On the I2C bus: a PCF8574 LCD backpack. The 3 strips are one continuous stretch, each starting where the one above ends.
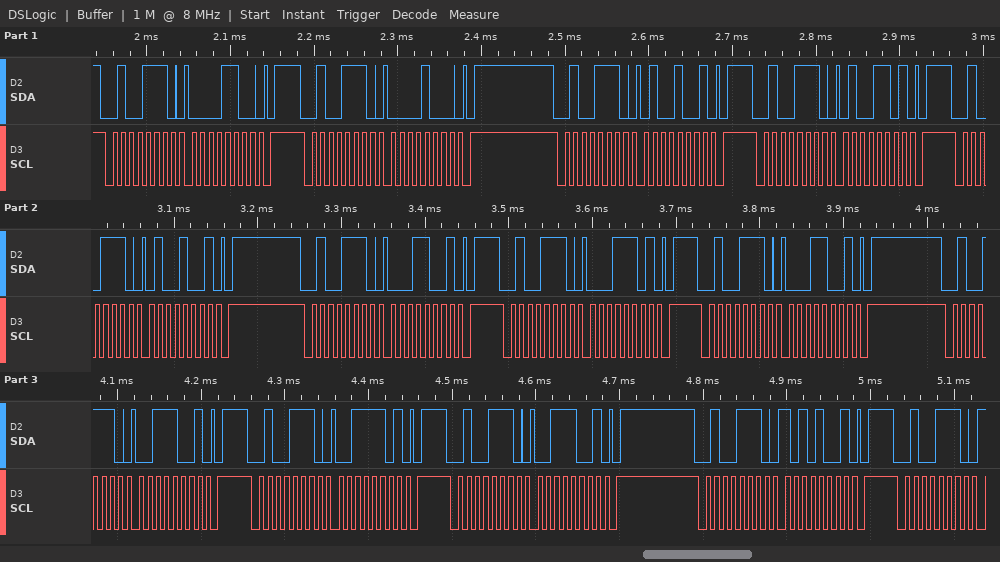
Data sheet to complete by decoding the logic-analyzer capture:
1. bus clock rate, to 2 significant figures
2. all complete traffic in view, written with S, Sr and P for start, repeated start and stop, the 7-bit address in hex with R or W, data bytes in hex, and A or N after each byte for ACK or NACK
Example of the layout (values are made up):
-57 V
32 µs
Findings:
100 kHz
S 27W A 0C A P S 27W A 08 A P S 27W A 49 A P S 27W A 4D A P S 27W A 49 A P S 27W A 19 A P S 27W A 1D A P S 27W A 19 A P S 27W A 39 A P S 27W A 3D A P S 27W A 39 A P S 27W A A9 A P S 27W A
